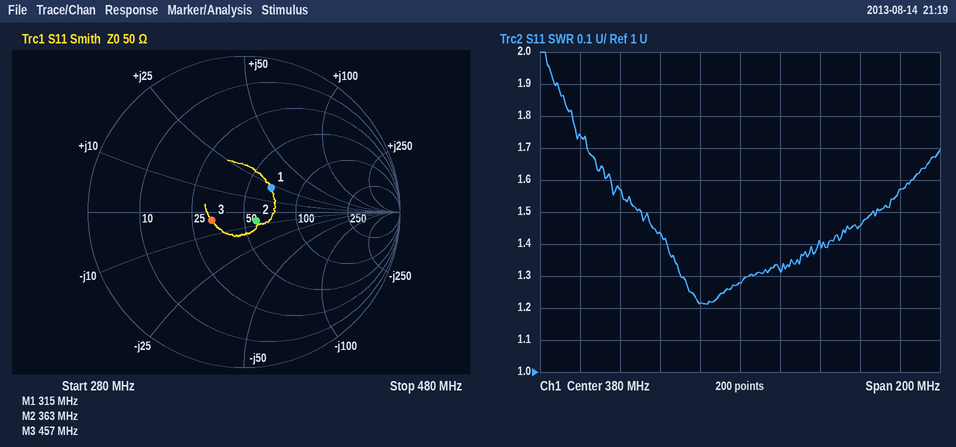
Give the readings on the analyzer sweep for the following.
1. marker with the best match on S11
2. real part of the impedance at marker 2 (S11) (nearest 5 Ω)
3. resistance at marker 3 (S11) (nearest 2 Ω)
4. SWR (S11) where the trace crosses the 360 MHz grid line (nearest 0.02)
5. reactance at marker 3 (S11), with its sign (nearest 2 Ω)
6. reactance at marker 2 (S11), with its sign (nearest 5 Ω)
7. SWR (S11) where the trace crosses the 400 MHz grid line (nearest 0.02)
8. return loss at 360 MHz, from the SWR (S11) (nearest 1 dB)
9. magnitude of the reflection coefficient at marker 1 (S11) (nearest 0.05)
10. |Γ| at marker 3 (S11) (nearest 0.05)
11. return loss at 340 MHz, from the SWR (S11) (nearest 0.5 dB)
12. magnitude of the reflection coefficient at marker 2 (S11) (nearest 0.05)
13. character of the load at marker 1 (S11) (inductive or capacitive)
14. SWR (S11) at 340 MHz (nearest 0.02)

marker 2
60 Ω
32 Ω
1.22
-4 Ω
-5 Ω
1.32
20 dB
0.25
0.20
15.0 dB
0.10
inductive
1.44
